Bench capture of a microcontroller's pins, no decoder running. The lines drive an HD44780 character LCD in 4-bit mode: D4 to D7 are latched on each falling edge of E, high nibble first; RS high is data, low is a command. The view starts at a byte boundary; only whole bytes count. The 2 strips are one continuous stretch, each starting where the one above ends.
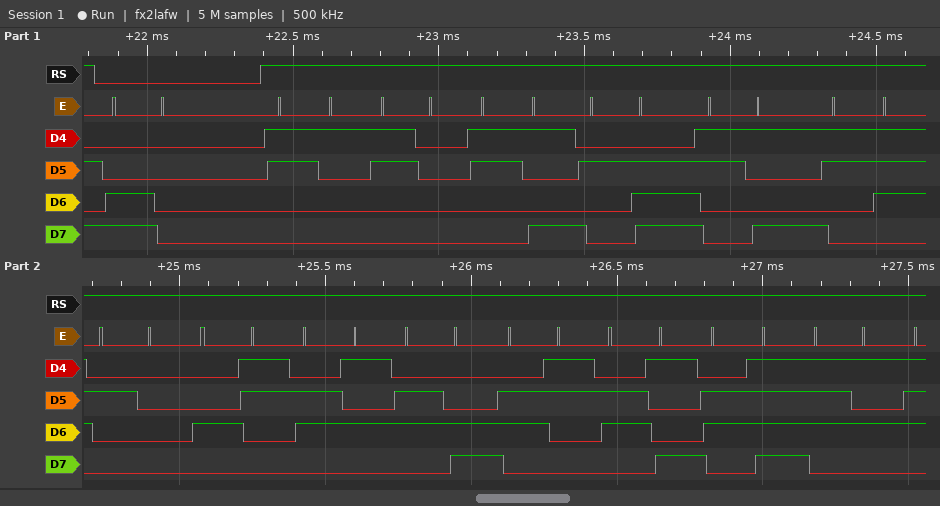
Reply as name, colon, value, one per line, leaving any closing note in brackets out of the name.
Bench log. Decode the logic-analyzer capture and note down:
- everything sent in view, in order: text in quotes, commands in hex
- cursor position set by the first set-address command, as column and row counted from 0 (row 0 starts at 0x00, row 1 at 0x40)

everything sent in view, in order: text in quotes, commands in hex: 0xC0 "109.97 Celciou"
cursor position set by the first set-address command, as column and row counted from 0: column 0, row 1
